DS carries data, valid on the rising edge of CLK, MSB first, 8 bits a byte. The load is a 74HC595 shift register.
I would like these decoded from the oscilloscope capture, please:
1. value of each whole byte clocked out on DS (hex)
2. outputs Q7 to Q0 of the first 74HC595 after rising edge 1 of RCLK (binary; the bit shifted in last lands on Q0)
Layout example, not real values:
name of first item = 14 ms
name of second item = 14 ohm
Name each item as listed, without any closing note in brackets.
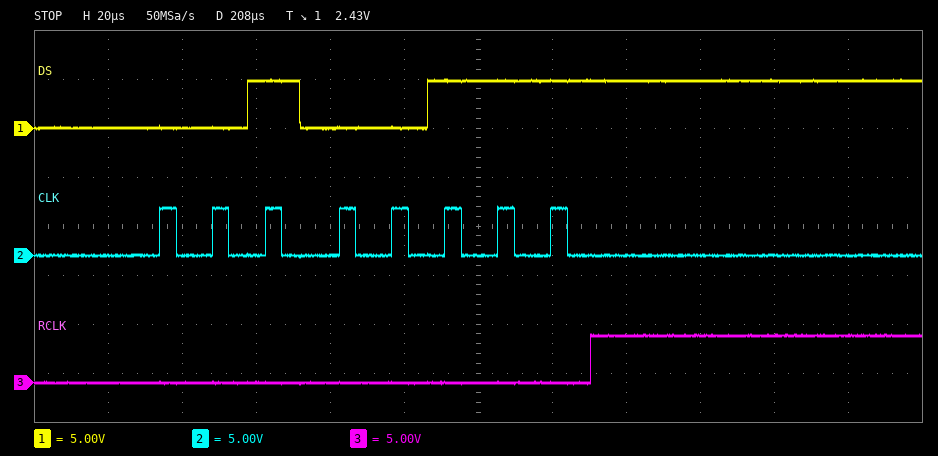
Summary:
value of each whole byte clocked out on DS = 27
outputs Q7 to Q0 of the first 74HC595 after rising edge 1 of RCLK = 00100111
